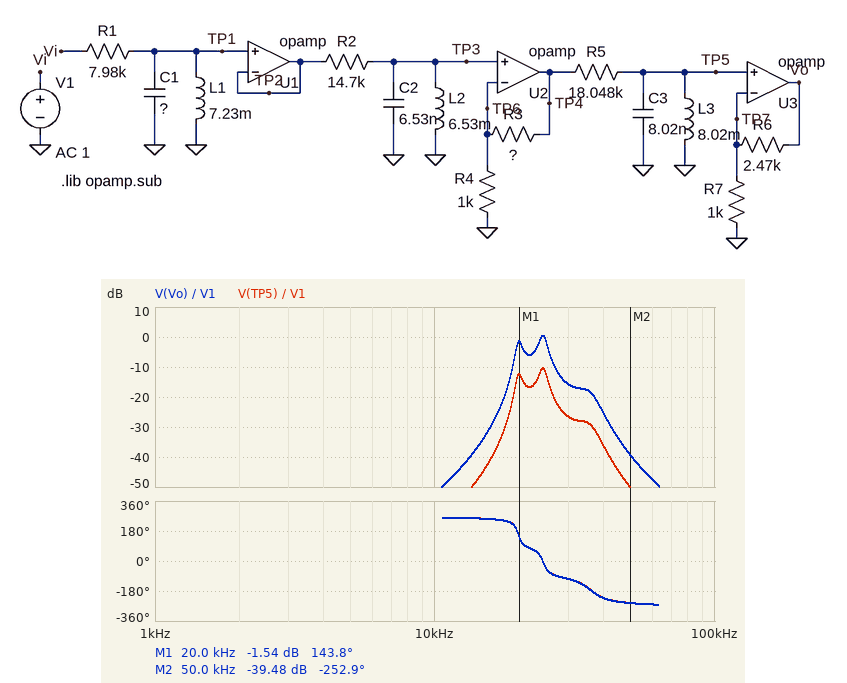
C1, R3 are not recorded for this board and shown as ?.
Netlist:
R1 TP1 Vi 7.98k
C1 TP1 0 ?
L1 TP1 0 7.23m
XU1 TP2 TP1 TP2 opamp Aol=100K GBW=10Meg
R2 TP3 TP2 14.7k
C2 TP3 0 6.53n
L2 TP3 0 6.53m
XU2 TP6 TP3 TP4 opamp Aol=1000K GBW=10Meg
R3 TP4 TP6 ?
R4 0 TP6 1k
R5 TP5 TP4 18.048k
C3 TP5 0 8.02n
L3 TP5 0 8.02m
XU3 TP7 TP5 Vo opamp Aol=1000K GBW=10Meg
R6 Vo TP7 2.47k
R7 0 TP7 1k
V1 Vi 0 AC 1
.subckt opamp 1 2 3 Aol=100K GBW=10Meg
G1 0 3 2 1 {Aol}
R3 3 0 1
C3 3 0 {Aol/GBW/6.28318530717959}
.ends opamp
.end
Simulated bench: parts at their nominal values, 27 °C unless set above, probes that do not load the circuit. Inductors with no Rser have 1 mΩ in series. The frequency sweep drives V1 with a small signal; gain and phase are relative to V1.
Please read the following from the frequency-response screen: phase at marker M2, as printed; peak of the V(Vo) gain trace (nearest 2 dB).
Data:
-252.9 deg
0 dB
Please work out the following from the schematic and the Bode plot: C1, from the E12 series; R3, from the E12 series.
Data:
2.7 nF
8.2 kΩ
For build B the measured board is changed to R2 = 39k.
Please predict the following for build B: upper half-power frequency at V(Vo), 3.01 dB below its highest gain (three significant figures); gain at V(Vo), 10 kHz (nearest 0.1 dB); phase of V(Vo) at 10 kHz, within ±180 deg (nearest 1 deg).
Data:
24.7 kHz
-60.6 dB
-97 deg
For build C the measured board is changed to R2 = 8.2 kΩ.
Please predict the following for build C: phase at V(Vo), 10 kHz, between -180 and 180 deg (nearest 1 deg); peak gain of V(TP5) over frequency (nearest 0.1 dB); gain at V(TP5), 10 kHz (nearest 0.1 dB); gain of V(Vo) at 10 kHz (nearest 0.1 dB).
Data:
-100 deg
-7.5 dB
-57.9 dB
-47.1 dB
